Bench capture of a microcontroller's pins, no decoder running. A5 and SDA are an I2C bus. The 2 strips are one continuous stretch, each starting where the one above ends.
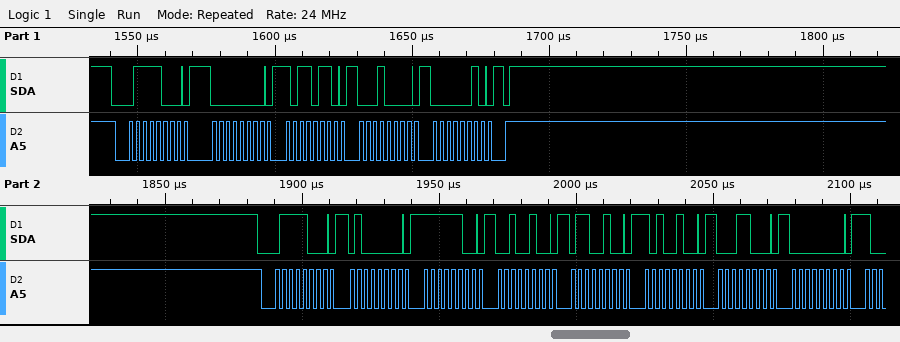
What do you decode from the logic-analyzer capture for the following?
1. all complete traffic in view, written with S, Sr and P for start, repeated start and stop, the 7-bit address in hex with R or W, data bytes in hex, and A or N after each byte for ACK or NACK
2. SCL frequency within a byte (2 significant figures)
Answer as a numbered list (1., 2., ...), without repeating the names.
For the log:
1. S 3CW A 00 A B6 A 10 A 02 A P S 3CW A 40 A FC A 24 A 64 A A4 A 18 A 00 A
2. 400 kHz
